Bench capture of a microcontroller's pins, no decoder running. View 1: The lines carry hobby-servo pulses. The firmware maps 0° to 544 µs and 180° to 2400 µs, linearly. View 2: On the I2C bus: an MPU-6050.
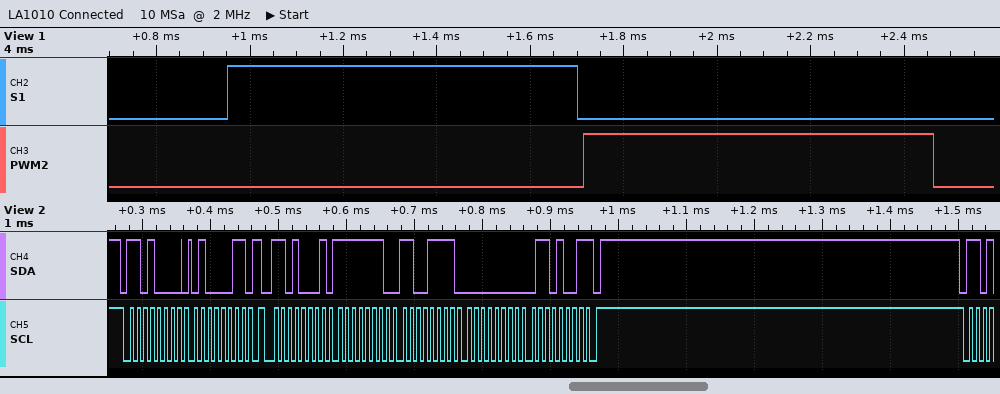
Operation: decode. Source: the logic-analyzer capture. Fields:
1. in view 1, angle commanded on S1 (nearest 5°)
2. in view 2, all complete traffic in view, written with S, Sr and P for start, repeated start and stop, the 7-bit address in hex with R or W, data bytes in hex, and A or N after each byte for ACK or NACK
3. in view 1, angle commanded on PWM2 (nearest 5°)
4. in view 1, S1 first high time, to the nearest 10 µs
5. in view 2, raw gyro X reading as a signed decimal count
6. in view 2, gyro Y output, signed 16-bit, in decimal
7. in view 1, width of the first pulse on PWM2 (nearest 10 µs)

20°
S 68W A 43 A Sr 68R A FE A CF A 00 A 69 N P
20°
750 µs
-305
105
750 µs
